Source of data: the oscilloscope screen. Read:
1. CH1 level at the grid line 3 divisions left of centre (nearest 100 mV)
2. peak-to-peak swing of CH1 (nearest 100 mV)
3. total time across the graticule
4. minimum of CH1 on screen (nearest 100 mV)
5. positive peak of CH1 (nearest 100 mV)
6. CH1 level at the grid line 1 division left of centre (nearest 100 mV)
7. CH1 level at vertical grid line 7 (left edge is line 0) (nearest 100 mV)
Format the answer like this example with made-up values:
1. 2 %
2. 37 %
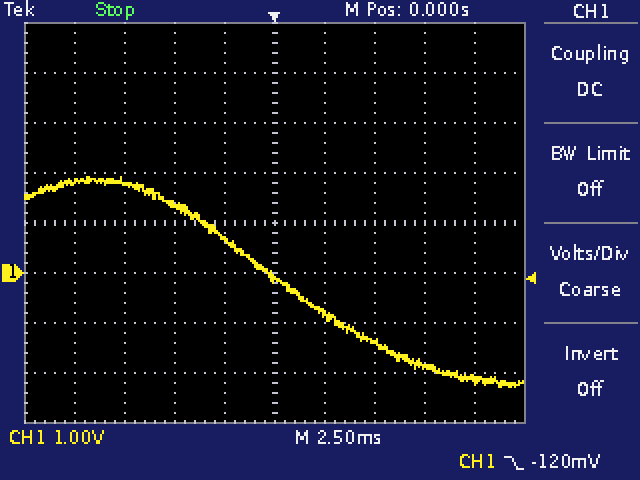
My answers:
1. 1.8 V
2. 4.2 V
3. 25 ms
4. -2.3 V
5. 1.9 V
6. 700 mV
7. -1.4 V
